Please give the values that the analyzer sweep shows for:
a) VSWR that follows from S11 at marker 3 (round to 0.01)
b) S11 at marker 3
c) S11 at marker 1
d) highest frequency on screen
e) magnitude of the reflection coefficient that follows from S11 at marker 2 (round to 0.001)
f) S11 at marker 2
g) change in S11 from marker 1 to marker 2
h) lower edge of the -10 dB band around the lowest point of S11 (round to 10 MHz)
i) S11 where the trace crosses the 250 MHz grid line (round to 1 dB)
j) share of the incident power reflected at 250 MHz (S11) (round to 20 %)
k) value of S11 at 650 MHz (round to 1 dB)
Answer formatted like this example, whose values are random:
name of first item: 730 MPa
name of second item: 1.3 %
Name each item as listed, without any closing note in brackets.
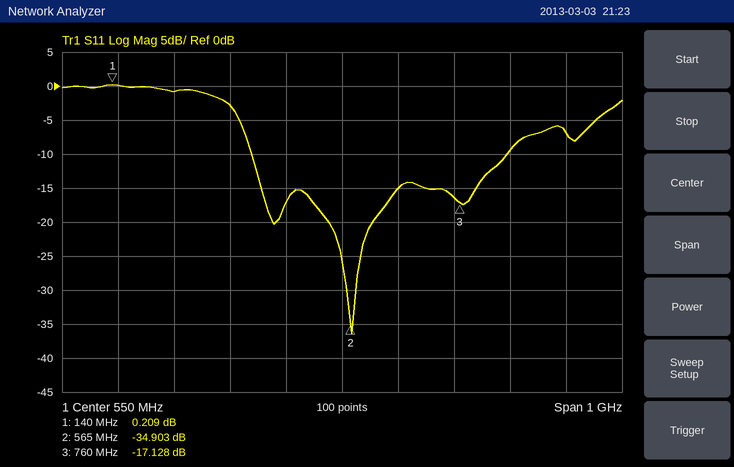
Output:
VSWR that follows from S11 at marker 3: 1.32
S11 at marker 3: -17.128 dB
S11 at marker 1: 0.209 dB
highest frequency on screen: 1.05 GHz
magnitude of the reflection coefficient that follows from S11 at marker 2: 0.018
S11 at marker 2: -34.903 dB
change in S11 from marker 1 to marker 2: -35.112 dB
lower edge of the -10 dB band around the lowest point of S11: 390 MHz
S11 where the trace crosses the 250 MHz grid line: -1 dB
share of the incident power reflected at 250 MHz (S11): 80 %
value of S11 at 650 MHz: -15 dB
